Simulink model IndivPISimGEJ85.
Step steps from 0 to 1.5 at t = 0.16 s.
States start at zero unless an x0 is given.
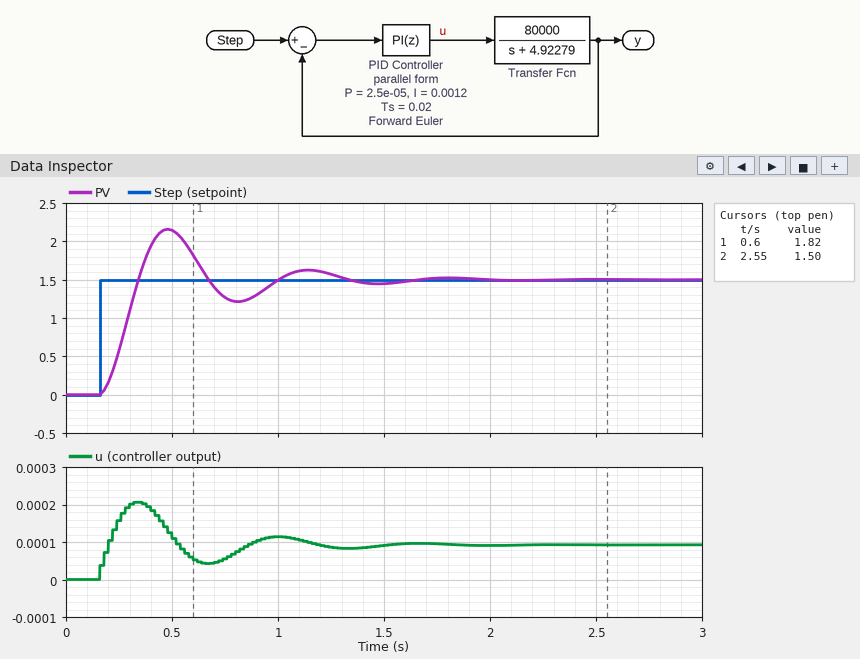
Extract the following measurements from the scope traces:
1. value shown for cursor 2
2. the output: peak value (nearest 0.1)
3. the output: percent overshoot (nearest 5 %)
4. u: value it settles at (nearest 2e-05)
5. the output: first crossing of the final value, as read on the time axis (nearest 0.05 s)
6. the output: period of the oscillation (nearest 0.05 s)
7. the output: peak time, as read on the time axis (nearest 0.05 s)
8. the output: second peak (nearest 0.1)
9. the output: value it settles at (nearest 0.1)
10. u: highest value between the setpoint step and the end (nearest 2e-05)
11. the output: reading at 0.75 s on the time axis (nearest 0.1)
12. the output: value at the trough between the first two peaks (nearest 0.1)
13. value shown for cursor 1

1.50
2.2
45 %
0.00010
0.35 s
0.65 s
0.50 s
1.6
1.5
0.00020
1.3
1.2
1.82
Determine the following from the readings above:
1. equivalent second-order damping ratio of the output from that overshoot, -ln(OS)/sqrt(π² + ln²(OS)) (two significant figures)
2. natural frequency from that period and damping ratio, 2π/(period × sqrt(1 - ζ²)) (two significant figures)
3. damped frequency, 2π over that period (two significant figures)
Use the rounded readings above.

0.25
10.0 rad/s
9.7 rad/s
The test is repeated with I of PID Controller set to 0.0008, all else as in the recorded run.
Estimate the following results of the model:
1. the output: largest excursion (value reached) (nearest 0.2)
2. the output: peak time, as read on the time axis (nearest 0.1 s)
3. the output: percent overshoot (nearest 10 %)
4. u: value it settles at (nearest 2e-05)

2.0
0.6 s
30 %
0.00010
